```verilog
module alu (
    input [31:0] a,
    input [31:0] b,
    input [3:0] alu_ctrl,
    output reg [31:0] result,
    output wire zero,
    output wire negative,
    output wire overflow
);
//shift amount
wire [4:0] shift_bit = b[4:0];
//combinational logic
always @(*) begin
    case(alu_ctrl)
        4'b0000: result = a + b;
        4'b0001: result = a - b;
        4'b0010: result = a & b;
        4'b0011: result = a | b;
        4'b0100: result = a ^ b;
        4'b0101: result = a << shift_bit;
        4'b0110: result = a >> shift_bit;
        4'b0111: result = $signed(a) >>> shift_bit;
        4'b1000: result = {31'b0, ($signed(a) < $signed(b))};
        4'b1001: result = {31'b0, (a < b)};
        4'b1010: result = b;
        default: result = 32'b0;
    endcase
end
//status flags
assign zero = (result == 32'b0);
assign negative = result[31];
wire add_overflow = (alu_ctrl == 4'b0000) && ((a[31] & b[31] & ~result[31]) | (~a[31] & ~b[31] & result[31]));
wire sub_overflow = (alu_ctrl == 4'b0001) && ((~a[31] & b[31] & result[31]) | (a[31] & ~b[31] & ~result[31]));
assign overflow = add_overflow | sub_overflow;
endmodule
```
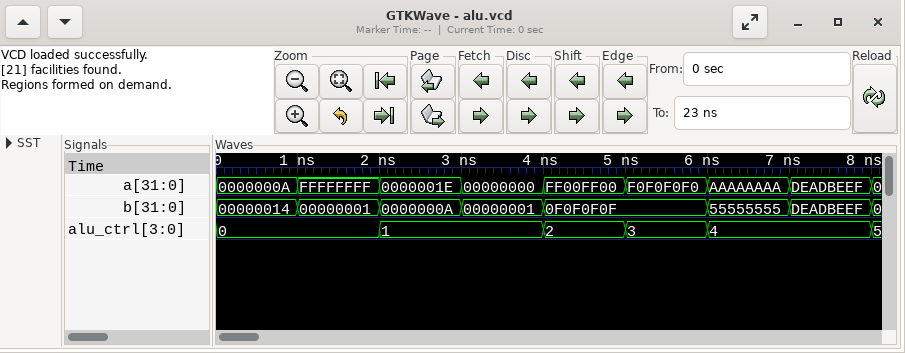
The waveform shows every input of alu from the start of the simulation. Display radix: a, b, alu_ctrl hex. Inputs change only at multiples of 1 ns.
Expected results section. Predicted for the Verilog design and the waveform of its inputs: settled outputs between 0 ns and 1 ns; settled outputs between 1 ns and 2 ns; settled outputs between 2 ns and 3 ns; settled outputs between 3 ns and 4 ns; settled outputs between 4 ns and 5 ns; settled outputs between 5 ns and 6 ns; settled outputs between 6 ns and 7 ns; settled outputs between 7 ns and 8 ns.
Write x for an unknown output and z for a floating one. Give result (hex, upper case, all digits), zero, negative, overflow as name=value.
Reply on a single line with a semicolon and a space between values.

result=0000001E, zero=0, negative=0, overflow=0; result=00000000, zero=1, negative=0, overflow=0; result=00000014, zero=0, negative=0, overflow=0; result=FFFFFFFF, zero=0, negative=1, overflow=0; result=0F000F00, zero=0, negative=0, overflow=0; result=FFFFFFFF, zero=0, negative=1, overflow=0; result=FFFFFFFF, zero=0, negative=1, overflow=0; result=00000000, zero=1, negative=0, overflow=0
